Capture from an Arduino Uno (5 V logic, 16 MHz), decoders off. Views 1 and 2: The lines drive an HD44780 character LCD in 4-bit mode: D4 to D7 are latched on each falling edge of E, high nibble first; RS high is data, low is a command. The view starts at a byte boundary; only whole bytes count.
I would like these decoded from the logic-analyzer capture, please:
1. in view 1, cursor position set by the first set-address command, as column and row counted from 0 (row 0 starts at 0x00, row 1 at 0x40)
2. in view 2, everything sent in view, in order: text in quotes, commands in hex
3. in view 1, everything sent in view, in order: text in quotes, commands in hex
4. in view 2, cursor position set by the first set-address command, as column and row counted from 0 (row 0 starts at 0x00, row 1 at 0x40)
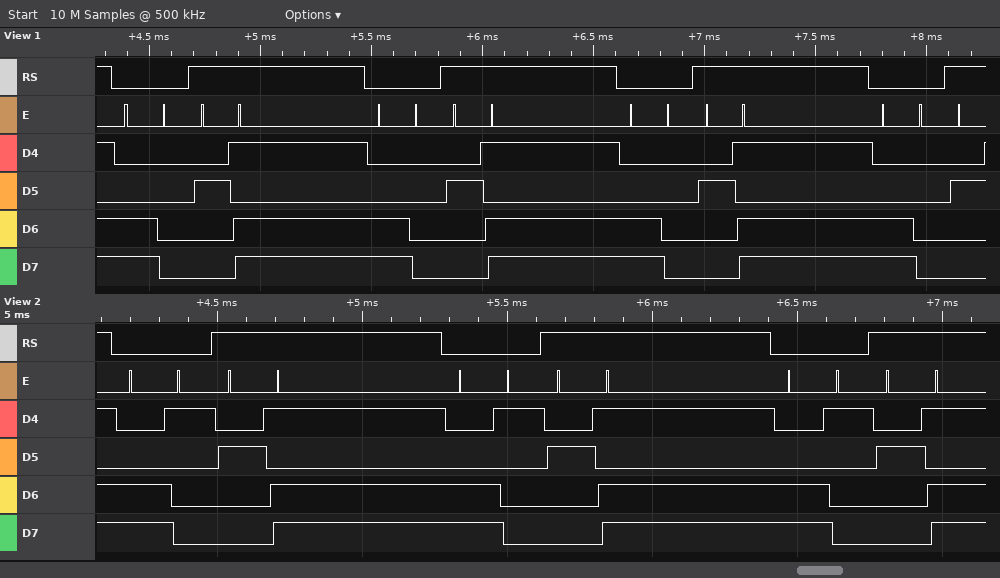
column 0, row 1
0xC1 "-" 0xC1 "-" 0xC1 "-"
0xC0 "-" 0xC0 "-" 0xC0 "-" 0xC0
column 1, row 1
